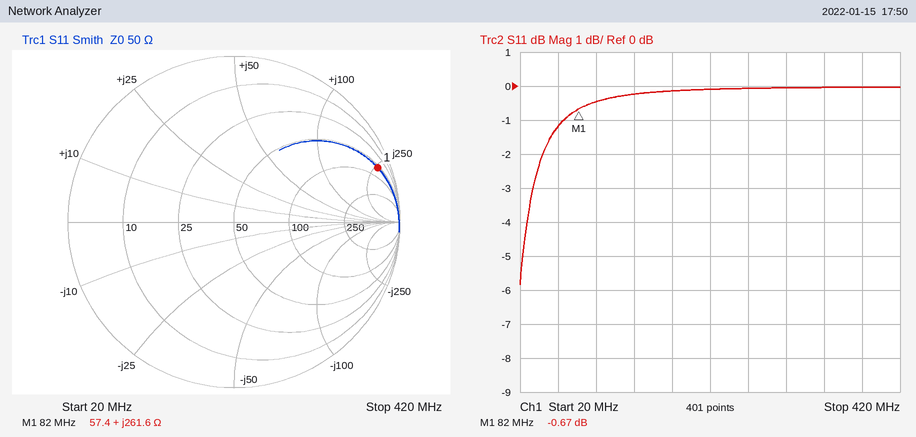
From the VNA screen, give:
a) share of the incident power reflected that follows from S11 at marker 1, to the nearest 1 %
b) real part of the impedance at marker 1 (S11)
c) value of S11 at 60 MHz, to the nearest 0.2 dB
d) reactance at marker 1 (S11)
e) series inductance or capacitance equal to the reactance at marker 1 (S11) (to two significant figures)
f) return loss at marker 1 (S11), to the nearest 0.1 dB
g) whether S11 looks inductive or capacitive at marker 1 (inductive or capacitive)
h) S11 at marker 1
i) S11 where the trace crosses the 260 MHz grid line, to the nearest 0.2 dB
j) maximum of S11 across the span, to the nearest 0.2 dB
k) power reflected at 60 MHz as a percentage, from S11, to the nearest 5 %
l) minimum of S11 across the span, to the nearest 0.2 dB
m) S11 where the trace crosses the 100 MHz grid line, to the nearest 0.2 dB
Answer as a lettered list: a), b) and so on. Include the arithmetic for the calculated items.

a) 10^(-0.67/10) ≈ 86 %
b) 57.4 Ω
c) -1.2 dB
d) +261.6 Ω
e) L = 261.6 Ω/(2π × 82 MHz) ≈ 508 nH, so 510 nH to two significant figures
f) 0.7 dB
g) inductive
h) -0.67 dB
i) 0.0 dB
j) 0.0 dB
k) 10^(-1.2/10) ≈ 75.9 %, so 75 % to the nearest 5 %
l) -5.8 dB
m) -0.4 dB
